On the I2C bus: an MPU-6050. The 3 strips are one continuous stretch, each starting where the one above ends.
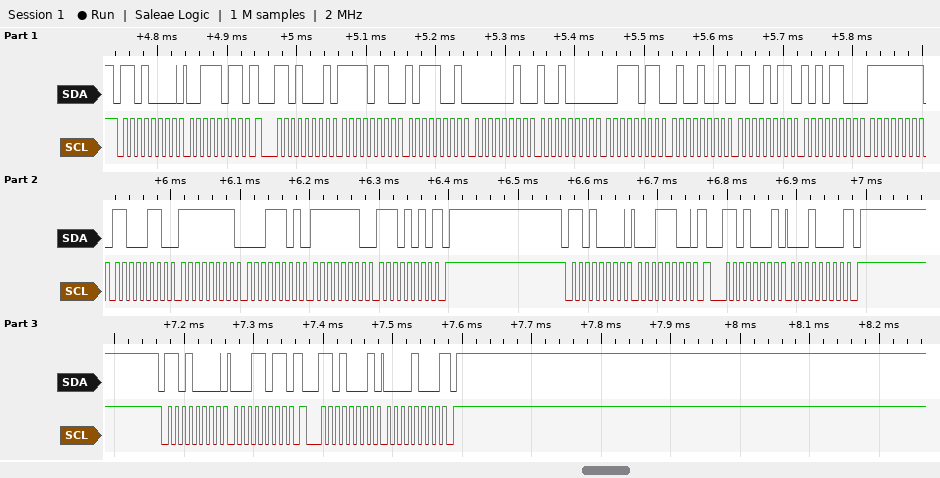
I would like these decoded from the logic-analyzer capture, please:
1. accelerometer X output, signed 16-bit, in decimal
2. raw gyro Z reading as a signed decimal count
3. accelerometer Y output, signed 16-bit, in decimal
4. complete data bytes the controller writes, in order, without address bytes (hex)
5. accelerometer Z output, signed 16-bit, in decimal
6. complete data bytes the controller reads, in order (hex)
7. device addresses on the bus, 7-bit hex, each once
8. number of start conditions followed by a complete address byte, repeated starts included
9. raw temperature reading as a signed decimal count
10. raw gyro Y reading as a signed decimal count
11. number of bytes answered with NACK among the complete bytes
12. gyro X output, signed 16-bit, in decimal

-2375
-278
656
3B 1C 1B
15177
F6 B9 02 90 3B 49 CB AC FF C6 FF 1D FE EA 10 08
0x68
6
-13396
-227
3
-58
